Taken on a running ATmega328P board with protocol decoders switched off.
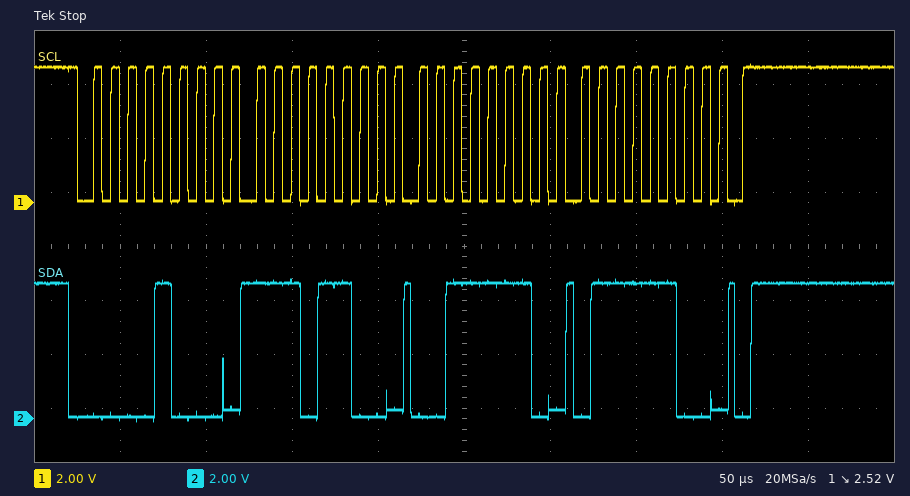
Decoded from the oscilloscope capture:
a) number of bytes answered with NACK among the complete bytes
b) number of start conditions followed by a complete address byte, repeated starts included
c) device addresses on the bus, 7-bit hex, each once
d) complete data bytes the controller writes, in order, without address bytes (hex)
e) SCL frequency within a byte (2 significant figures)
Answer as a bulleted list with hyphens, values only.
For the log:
- 0
- 1
- 0x04
- EC 3E 7C
- 100 kHz
